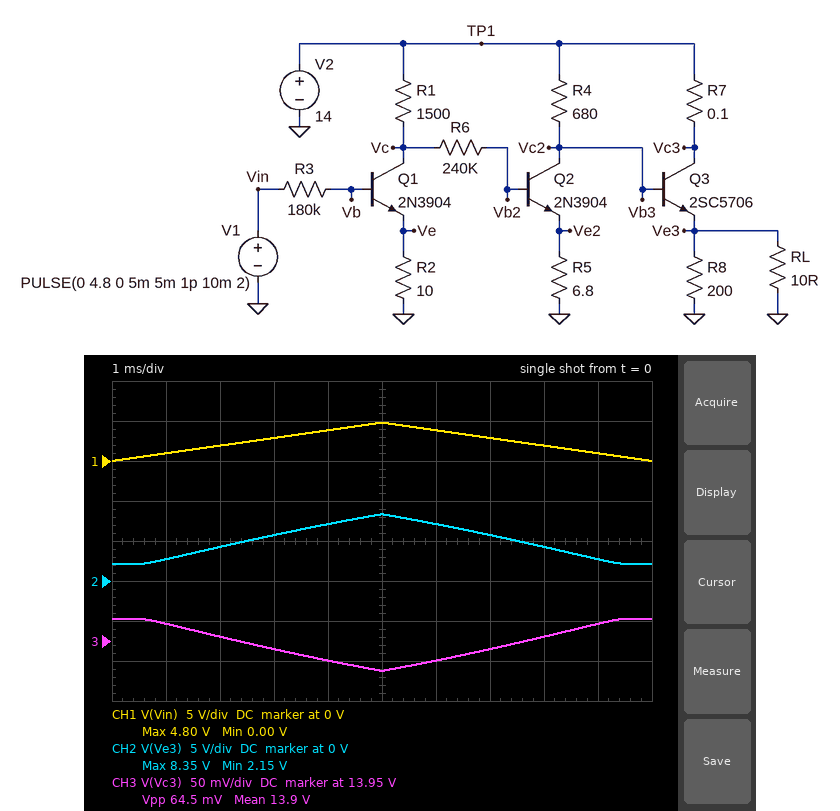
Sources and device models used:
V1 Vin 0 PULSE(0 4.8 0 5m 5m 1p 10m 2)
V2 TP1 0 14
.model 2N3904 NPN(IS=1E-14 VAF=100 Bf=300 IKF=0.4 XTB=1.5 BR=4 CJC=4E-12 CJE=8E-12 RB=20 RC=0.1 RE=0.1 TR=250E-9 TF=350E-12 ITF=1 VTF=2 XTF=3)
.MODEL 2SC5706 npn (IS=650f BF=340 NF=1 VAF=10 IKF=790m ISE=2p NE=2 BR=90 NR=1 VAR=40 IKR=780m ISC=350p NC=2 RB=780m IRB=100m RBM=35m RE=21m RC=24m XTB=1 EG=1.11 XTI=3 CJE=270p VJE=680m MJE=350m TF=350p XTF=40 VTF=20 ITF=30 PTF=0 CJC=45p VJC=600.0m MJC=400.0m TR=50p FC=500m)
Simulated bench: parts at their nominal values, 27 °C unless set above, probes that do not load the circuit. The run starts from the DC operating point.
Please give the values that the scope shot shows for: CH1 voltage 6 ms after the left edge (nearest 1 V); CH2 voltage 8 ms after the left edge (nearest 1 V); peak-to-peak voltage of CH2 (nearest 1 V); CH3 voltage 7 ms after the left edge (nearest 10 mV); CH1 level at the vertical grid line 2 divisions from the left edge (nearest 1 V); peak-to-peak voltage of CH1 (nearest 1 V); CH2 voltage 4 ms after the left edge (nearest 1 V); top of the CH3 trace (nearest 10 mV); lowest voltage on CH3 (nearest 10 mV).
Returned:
4 V
4 V
6 V
13.94 V
2 V
5 V
7 V
13.98 V
13.91 V
